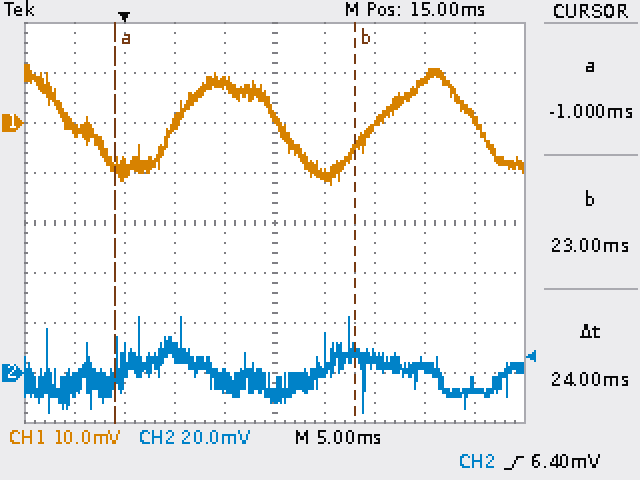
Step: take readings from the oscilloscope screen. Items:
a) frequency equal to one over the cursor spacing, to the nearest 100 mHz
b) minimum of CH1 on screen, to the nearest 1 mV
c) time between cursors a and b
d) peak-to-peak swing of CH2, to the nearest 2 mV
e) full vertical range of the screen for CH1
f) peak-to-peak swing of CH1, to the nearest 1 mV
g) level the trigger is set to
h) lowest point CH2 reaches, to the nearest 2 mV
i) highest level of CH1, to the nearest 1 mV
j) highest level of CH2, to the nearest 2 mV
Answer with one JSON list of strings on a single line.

["41.7 Hz", "-12 mV", "24 ms", "38 mV", "80 mV", "24 mV", "6.40 mV", "-16 mV", "12 mV", "22 mV"]
